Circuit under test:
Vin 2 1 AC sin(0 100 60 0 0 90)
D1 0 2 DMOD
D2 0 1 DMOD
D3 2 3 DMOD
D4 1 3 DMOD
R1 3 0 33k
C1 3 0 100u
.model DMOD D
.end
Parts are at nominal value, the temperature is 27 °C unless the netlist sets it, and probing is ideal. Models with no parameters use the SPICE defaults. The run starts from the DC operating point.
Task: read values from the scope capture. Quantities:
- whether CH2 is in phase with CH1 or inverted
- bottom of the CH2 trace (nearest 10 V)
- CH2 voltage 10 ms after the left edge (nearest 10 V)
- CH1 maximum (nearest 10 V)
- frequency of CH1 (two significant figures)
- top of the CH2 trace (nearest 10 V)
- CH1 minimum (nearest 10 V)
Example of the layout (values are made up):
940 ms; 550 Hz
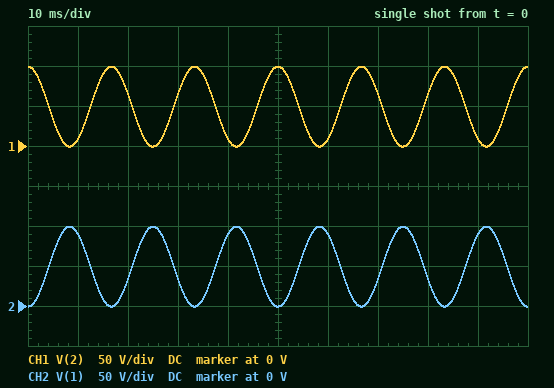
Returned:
inverted; 0 V; 90 V; 100 V; 60 Hz; 100 V; 0 V
